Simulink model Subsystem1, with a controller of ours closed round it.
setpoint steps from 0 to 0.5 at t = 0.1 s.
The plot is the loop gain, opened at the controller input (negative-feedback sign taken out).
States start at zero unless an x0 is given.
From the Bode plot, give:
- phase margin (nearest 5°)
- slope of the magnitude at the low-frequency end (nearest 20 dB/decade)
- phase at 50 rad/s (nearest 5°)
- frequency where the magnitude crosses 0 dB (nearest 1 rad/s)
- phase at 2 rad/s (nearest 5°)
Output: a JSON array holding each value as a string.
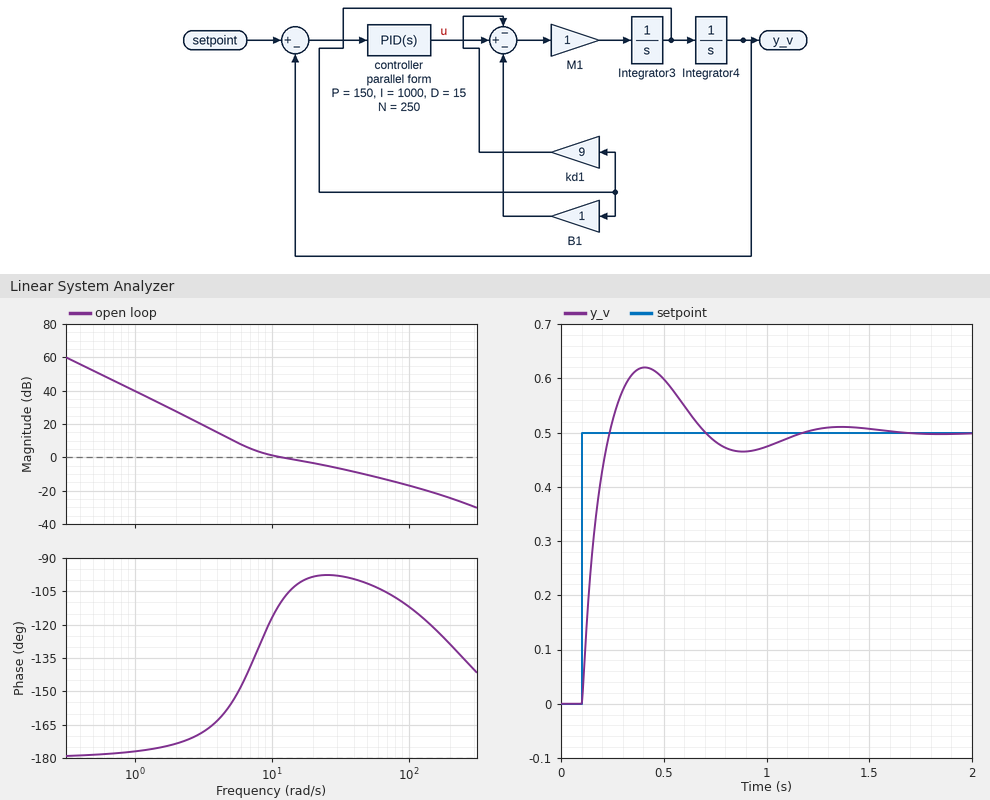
["70°", "-40 dB/decade", "-100°", "12 rad/s", "-175°"]
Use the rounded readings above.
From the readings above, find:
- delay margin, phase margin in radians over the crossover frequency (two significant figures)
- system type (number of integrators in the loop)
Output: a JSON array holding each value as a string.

["0.10 s", "2"]
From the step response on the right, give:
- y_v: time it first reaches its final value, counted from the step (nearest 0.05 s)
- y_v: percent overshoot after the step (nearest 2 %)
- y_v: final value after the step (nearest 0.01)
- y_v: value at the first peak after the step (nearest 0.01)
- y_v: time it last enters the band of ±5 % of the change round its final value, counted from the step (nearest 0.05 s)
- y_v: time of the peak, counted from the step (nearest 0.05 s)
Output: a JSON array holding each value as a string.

["0.15 s", "24 %", "0.50", "0.62", "0.90 s", "0.30 s"]
